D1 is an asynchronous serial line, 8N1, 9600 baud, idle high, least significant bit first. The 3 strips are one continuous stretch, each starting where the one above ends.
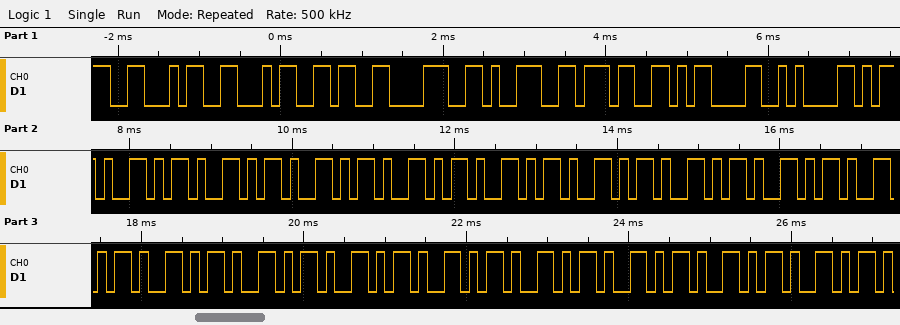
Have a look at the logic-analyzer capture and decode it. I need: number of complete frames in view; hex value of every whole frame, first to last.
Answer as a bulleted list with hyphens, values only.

- 25
- 46 46 36 38 39 37 0D 0A 2D 2D 2D 2D 2D 2D 2D 2D 2D 2D 2D 2D 2D 2D 2D 2D 2D
